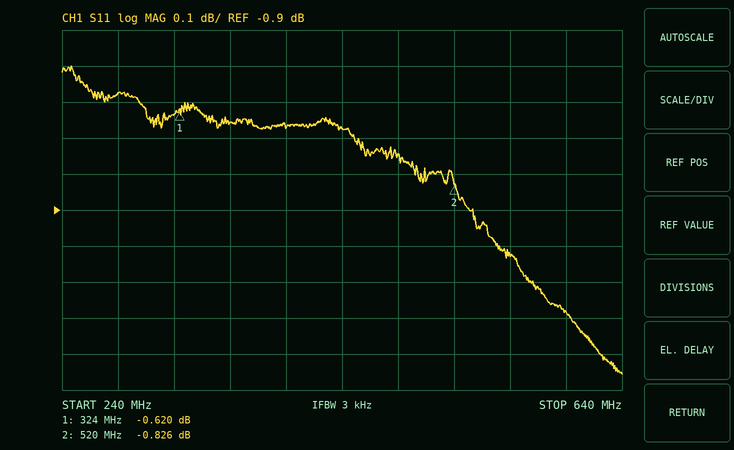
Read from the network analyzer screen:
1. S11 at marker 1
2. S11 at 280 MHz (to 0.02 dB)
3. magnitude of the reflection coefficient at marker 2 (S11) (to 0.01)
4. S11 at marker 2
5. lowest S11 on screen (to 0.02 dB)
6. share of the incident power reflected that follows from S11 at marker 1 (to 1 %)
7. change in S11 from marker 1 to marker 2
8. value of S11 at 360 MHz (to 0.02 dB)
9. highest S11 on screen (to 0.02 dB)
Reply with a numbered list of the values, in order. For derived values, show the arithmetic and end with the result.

1. -0.620 dB
2. -0.58 dB
3. 10^(-0.826/20) ≈ 0.91
4. -0.826 dB
5. -1.36 dB
6. 10^(-0.62/10) ≈ 87 %
7. -0.826 − (-0.62) = -0.206 dB
8. -0.66 dB
9. -0.50 dB
